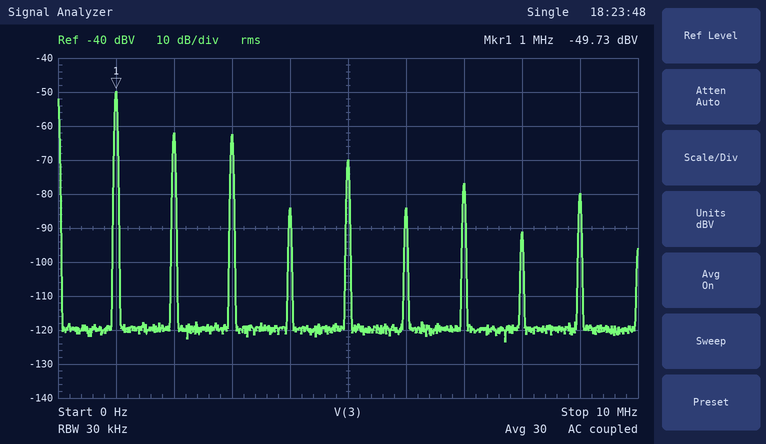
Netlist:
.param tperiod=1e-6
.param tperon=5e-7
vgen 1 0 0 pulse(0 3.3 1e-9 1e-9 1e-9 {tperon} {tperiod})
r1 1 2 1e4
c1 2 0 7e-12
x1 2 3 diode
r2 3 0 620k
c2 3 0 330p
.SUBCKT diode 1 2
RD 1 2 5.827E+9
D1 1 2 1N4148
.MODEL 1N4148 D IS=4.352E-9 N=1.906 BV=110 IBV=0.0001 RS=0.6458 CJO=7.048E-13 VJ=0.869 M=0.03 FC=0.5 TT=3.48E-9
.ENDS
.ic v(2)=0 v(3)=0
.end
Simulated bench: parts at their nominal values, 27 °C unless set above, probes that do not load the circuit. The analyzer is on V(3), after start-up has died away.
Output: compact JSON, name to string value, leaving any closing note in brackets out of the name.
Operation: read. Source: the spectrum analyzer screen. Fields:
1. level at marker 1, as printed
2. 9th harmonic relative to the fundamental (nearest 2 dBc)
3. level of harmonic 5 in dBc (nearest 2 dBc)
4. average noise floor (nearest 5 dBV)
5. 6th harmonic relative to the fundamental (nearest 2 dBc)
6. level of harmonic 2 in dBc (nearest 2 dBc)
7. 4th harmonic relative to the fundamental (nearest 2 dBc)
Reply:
{"level at marker 1, as printed": "-49.73 dBV", "9th harmonic relative to the fundamental": "-30 dBc", "level of harmonic 5 in dBc": "-20 dBc", "average noise floor": "-120 dBV", "6th harmonic relative to the fundamental": "-34 dBc", "level of harmonic 2 in dBc": "-12 dBc", "4th harmonic relative to the fundamental": "-34 dBc"}
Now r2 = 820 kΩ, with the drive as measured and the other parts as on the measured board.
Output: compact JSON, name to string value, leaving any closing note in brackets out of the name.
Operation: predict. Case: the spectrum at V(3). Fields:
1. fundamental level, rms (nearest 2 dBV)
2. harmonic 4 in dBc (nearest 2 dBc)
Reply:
{"fundamental level, rms": "-50 dBV", "harmonic 4 in dBc": "-38 dBc"}
